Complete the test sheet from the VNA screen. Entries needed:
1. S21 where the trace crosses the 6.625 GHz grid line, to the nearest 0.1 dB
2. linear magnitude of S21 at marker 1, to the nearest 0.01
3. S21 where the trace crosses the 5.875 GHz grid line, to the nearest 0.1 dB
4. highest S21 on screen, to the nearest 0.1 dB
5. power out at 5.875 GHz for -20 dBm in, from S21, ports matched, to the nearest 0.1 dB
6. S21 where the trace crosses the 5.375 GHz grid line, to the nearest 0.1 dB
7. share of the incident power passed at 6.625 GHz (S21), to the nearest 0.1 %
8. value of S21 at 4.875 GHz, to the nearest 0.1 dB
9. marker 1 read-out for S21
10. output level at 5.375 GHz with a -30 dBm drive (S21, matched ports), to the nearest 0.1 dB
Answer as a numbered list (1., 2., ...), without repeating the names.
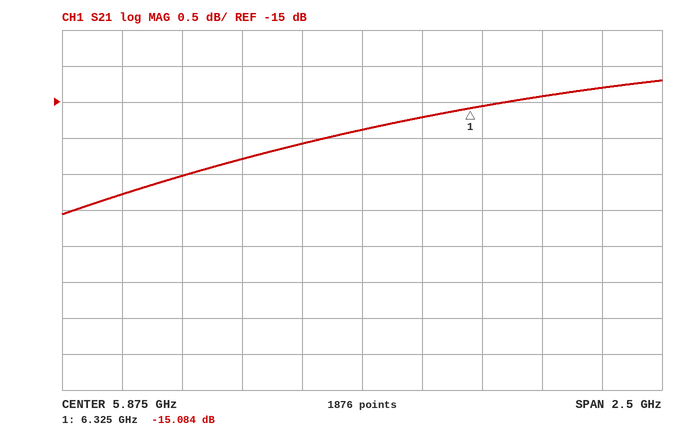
1. -14.9 dB
2. 0.18
3. -15.4 dB
4. -14.7 dB
5. -35.4 dBm
6. -15.8 dB
7. 3.2 %
8. -16.3 dB
9. -15.084 dB
10. -45.8 dBm
